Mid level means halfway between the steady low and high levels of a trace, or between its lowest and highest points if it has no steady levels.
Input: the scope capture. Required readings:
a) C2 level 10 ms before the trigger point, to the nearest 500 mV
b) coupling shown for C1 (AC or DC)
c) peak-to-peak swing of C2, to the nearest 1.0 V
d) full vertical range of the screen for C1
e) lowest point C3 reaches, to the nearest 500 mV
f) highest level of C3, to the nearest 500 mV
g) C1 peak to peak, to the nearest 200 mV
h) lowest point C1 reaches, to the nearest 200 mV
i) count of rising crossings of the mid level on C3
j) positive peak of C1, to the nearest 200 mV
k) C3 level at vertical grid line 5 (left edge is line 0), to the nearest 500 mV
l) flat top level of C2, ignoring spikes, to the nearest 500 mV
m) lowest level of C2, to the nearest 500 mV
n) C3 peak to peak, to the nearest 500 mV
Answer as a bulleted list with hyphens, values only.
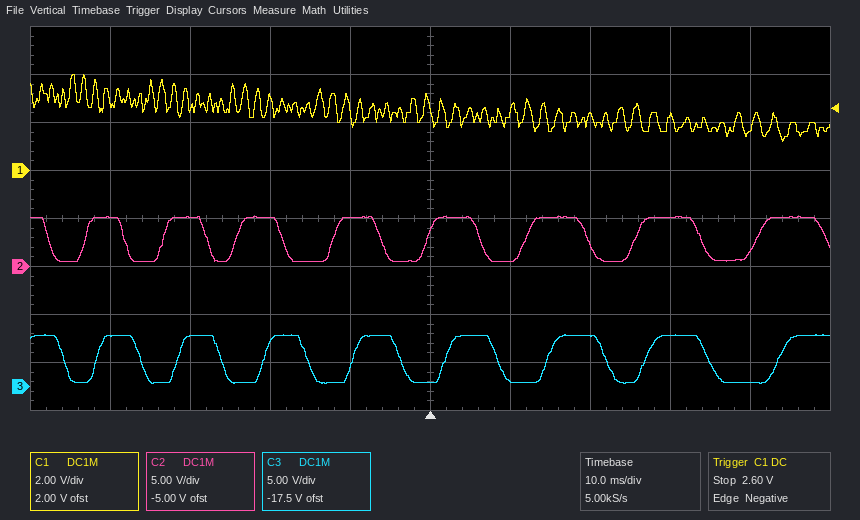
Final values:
- 5.0 V
- DC
- 5.0 V
- 16 V
- 500 mV
- 5.5 V
- 2.8 V
- 1.2 V
- 8
- 4.0 V
- 500 mV
- 5.0 V
- 500 mV
- 5.0 V
